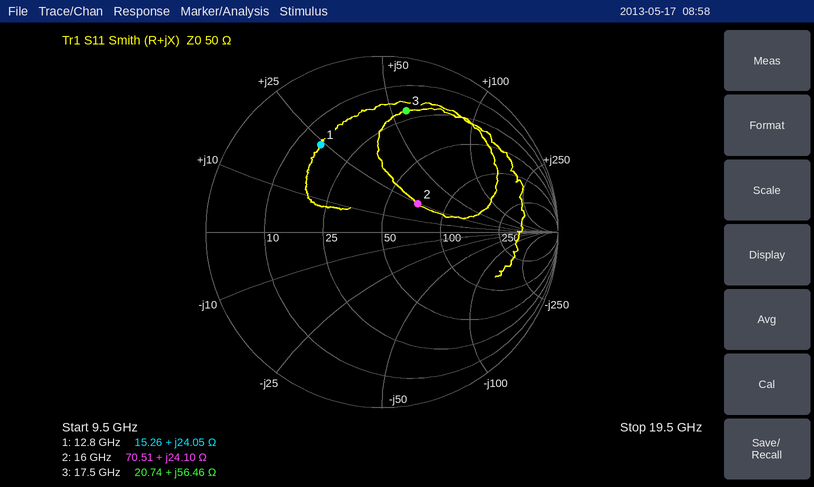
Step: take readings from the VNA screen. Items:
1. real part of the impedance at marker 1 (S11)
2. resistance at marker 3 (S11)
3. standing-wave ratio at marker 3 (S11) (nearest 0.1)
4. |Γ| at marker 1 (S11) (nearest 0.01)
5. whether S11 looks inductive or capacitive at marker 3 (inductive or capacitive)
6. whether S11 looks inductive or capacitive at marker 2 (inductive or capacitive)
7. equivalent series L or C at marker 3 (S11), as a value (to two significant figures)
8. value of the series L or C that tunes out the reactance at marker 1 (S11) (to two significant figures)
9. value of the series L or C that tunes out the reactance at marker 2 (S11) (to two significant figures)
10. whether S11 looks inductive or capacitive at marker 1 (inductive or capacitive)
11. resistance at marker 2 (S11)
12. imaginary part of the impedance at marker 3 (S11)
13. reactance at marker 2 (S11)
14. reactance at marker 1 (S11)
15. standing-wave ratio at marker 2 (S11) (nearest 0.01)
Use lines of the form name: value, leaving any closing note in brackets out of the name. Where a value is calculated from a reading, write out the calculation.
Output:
real part of the impedance at marker 1: 15.26 Ω
resistance at marker 3: 20.74 Ω
standing-wave ratio at marker 3 (S11): 5.7
|Γ| at marker 1 (S11): 0.61
whether S11 looks inductive or capacitive at marker 3: inductive
whether S11 looks inductive or capacitive at marker 2: inductive
equivalent series L or C at marker 3 (S11), as a value: L = 56.46 Ω/(2π × 17.5 GHz) ≈ 513 pH, so 510 pH to two significant figures
value of the series L or C that tunes out the reactance at marker 1 (S11): C = 1/(2π × 12.8 GHz × 24.05 Ω) ≈ 517 fF, so 520 fF to two significant figures
value of the series L or C that tunes out the reactance at marker 2 (S11): C = 1/(2π × 16 GHz × 24.1 Ω) ≈ 413 fF, so 410 fF to two significant figures
whether S11 looks inductive or capacitive at marker 1: inductive
resistance at marker 2: 70.51 Ω
imaginary part of the impedance at marker 3: +56.46 Ω
reactance at marker 2: +24.10 Ω
reactance at marker 1: +24.05 Ω
standing-wave ratio at marker 2 (S11): 1.69
